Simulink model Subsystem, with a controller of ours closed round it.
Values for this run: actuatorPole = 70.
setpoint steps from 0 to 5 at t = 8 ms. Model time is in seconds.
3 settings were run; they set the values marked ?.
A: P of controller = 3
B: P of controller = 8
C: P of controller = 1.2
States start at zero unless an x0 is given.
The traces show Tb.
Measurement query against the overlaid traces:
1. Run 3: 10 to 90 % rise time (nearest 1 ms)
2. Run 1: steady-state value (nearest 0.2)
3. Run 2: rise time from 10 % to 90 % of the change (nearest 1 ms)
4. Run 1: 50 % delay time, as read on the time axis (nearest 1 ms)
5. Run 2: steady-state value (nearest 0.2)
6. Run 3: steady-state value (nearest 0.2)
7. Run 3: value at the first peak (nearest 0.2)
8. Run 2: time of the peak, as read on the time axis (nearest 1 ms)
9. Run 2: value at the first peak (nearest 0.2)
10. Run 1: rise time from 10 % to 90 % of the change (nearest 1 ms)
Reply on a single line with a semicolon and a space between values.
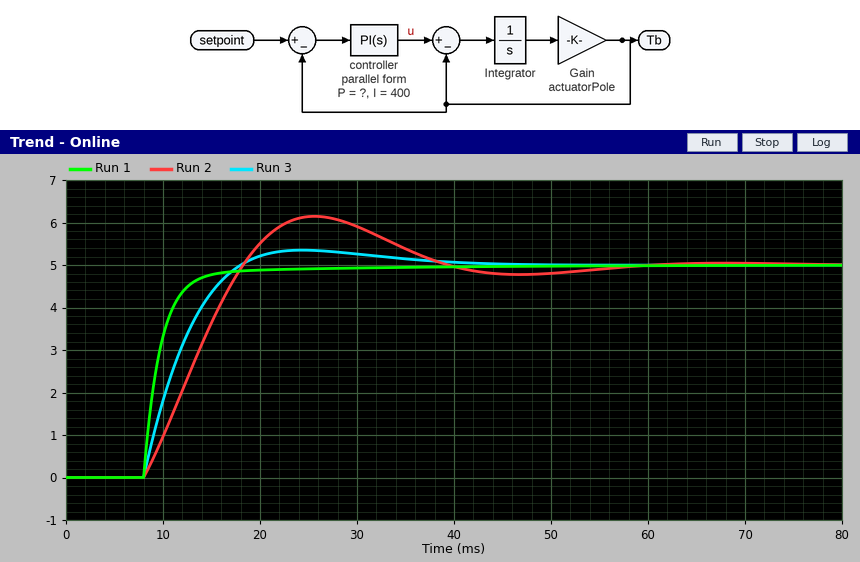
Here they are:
7 ms; 5.0; 8 ms; 9 ms; 5.0; 5.0; 5.4; 26 ms; 6.2; 4 ms
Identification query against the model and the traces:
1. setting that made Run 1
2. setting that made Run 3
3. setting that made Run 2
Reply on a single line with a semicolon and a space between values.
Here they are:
B; A; C
